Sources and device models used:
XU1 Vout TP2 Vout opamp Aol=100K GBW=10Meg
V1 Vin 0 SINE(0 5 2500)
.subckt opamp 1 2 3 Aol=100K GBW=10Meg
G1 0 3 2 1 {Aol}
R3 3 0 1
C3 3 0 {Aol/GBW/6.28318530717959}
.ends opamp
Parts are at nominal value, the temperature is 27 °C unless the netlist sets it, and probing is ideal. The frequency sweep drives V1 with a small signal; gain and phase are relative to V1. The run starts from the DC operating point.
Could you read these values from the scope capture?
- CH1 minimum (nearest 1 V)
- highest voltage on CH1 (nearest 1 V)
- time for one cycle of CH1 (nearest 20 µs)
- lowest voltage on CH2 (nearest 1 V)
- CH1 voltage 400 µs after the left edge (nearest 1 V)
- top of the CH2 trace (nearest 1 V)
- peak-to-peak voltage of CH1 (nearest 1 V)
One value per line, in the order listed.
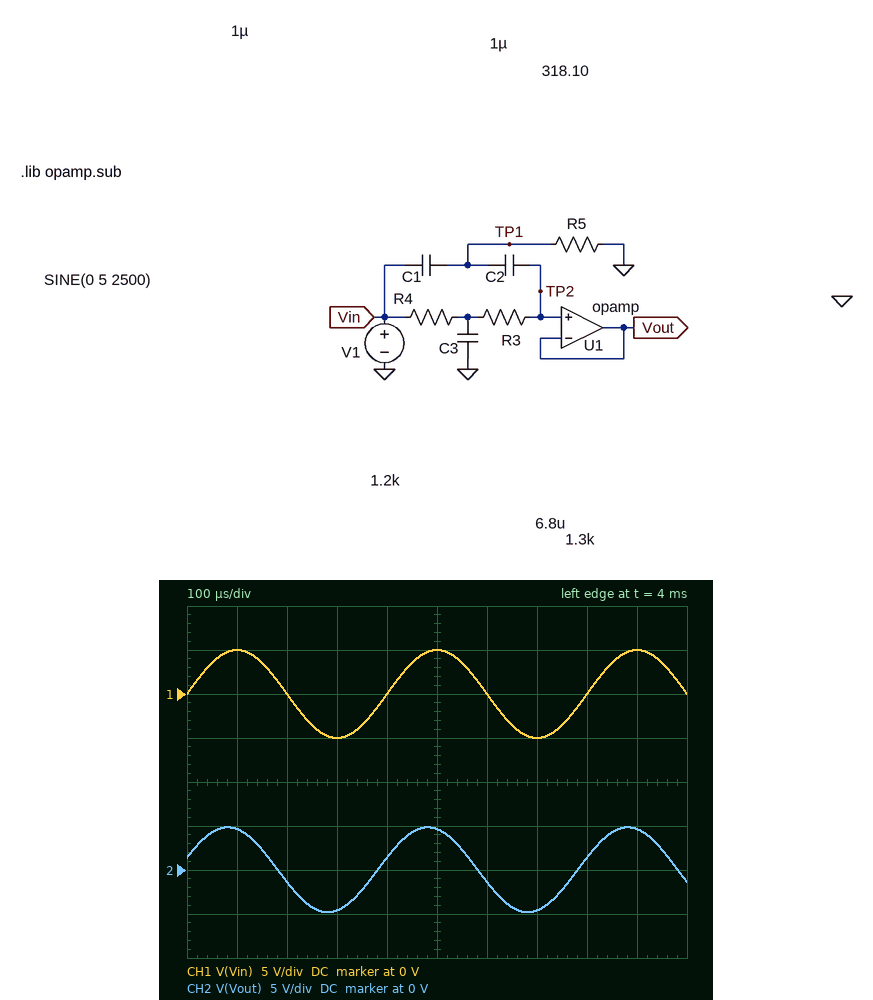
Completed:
-5 V
5 V
400 µs
-5 V
0 V
5 V
10 V
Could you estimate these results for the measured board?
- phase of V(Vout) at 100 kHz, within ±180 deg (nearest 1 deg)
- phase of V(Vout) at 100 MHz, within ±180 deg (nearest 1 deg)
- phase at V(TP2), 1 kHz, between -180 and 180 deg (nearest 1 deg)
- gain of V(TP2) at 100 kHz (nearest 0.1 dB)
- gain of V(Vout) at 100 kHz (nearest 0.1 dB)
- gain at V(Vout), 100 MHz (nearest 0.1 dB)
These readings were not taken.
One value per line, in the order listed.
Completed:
0 deg
-84 deg
38 deg
0 dB
0 dB
-20.0 dB
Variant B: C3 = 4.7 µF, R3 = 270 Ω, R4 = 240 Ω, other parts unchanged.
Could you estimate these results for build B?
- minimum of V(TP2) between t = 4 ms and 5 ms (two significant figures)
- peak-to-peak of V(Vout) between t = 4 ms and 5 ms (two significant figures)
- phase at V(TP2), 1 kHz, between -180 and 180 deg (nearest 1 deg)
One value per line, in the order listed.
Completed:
-4.1 V
8.2 V
63 deg
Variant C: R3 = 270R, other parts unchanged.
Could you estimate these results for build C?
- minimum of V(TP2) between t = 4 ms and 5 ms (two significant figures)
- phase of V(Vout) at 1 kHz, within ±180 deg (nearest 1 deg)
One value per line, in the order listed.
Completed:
-4.2 V
65 deg
